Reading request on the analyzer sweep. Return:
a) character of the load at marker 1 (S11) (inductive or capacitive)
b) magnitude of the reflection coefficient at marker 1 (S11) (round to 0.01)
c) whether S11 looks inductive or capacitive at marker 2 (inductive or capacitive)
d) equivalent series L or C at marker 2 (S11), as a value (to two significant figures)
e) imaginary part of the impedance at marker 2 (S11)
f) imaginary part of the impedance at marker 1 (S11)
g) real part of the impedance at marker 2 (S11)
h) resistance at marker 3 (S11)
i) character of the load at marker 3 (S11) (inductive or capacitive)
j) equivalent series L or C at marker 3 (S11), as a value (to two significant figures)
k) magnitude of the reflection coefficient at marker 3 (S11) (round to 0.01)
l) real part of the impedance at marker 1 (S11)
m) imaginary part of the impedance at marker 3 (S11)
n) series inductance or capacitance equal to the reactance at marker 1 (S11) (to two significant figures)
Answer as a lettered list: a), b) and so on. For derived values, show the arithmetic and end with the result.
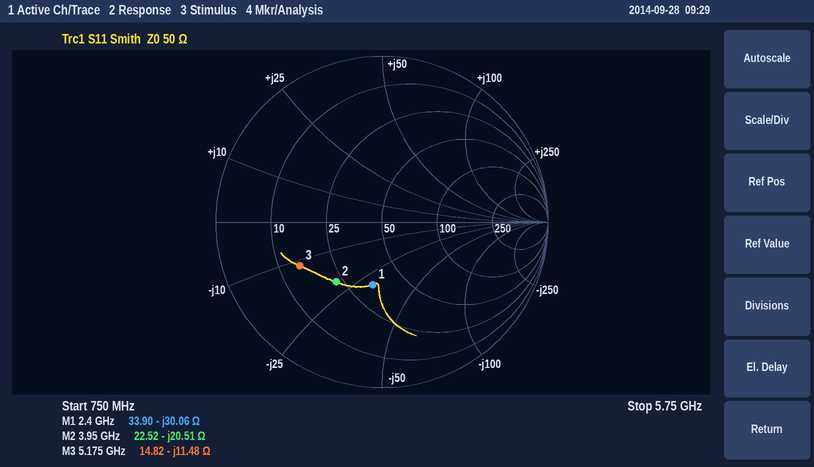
a) capacitive
b) 0.38
c) capacitive
d) C = 1/(2π × 3.95 GHz × 20.51 Ω) ≈ 2.0 pF
e) -20.51 Ω
f) -30.06 Ω
g) 22.52 Ω
h) 14.82 Ω
i) capacitive
j) C = 1/(2π × 5.175 GHz × 11.48 Ω) ≈ 2.7 pF
k) 0.56
l) 33.90 Ω
m) -11.48 Ω
n) C = 1/(2π × 2.4 GHz × 30.06 Ω) ≈ 2.2 pF
